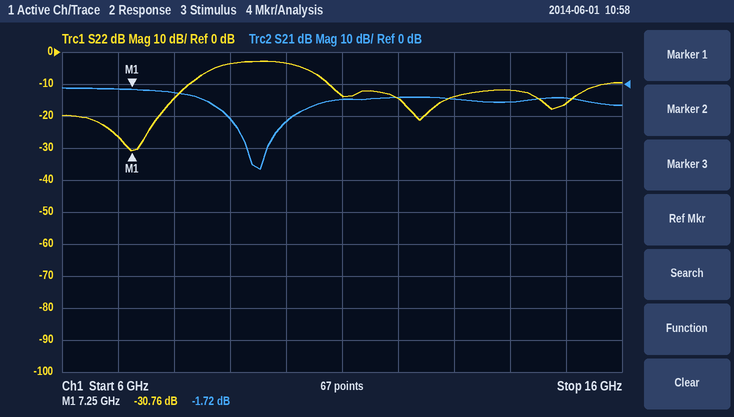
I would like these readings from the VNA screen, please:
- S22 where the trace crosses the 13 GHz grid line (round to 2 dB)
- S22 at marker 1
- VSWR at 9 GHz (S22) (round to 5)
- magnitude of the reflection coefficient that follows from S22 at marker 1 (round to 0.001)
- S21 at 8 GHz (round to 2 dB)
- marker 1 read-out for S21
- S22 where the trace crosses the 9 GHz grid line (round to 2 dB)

-14 dB
-30.76 dB
5
0.029
-2 dB
-1.72 dB
-4 dB
